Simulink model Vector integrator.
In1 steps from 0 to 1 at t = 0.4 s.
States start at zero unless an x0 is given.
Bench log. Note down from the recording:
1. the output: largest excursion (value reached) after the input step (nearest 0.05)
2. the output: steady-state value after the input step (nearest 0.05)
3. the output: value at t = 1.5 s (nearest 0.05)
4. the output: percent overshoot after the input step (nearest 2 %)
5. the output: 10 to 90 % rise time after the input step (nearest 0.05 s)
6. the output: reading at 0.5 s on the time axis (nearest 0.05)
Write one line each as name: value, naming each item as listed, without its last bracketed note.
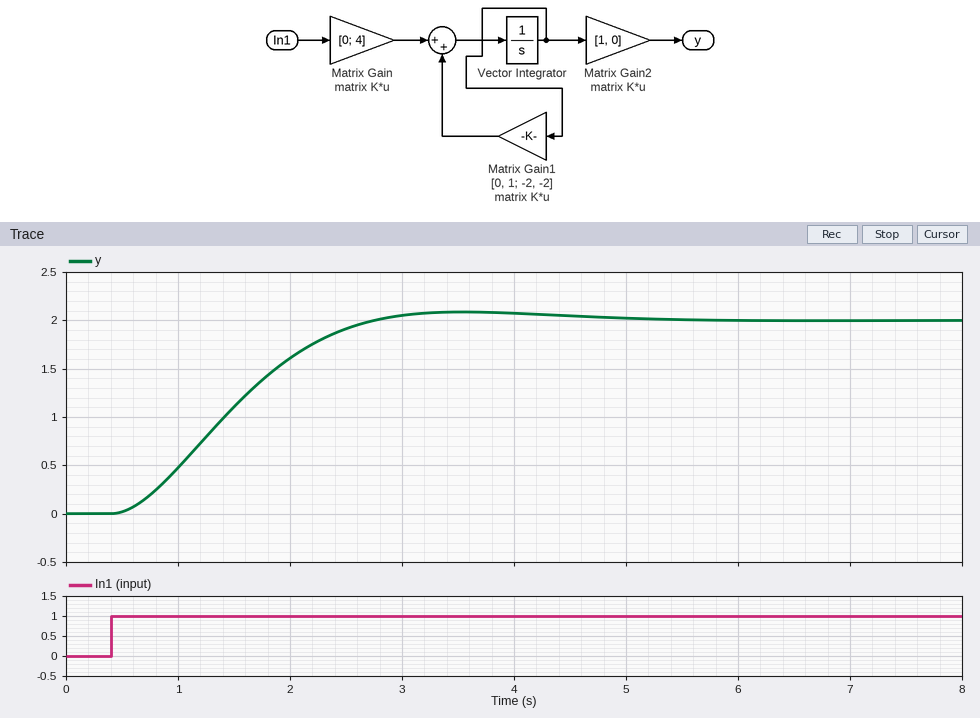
the output: largest excursion (value reached) after the input step: 2.10
the output: steady-state value after the input step: 2.00
the output: value at t = 1.5 s: 1.10
the output: percent overshoot after the input step: 4 %
the output: 10 to 90 % rise time after the input step: 1.50 s
the output: reading at 0.5 s on the time axis: 0.00
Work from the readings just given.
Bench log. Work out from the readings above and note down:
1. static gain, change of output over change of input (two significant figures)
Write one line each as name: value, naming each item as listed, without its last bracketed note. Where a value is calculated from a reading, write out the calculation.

static gain, change of output over change of input: (2 - 0) / (1 - 0) = 2.0
